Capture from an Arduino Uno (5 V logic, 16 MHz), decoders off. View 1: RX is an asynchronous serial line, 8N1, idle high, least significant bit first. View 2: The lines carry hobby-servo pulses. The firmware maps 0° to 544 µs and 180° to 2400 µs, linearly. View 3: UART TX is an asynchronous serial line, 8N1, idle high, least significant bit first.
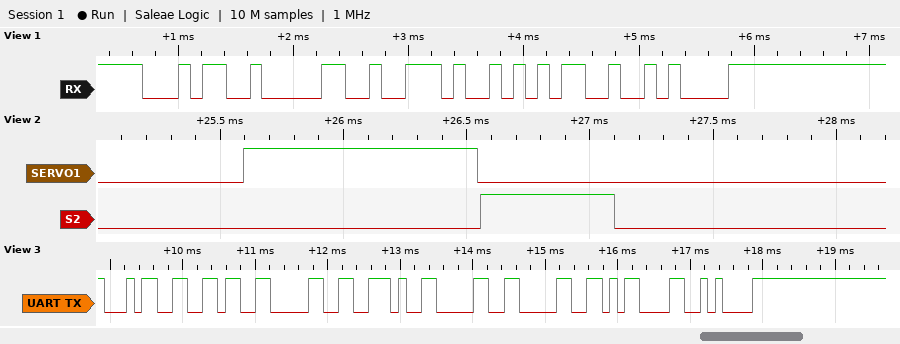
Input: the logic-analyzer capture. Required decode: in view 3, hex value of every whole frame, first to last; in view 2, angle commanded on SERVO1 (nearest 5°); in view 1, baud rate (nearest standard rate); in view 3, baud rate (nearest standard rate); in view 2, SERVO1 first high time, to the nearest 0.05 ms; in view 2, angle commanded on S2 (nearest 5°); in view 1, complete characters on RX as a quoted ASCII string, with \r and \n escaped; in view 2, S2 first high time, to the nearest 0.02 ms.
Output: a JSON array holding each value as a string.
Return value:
["0x34 0x36 0x30 0x2E 0x30 0x30 0x0D 0x0A", "40°", "9600 baud", "9600 baud", "0.95 ms", "0°", "\"40.5\\n\"", "0.54 ms"]
